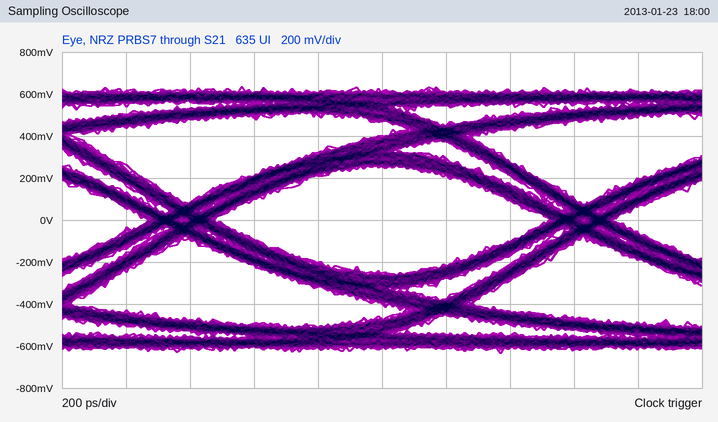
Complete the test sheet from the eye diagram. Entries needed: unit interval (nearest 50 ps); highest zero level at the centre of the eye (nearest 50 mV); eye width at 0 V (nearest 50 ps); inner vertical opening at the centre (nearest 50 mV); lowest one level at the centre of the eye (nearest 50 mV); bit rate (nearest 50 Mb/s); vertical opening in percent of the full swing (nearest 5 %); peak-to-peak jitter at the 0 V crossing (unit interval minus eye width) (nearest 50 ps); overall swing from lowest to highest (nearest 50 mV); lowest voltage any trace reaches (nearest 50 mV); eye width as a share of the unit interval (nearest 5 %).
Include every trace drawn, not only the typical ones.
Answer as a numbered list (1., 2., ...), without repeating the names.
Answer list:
1. 1.25 ns
2. -250 mV
3. 1.05 ns
4. 500 mV
5. 250 mV
6. 800 Mb/s
7. 40 %
8. 200 ps
9. 1.25 V
10. -650 mV
11. 85 %
